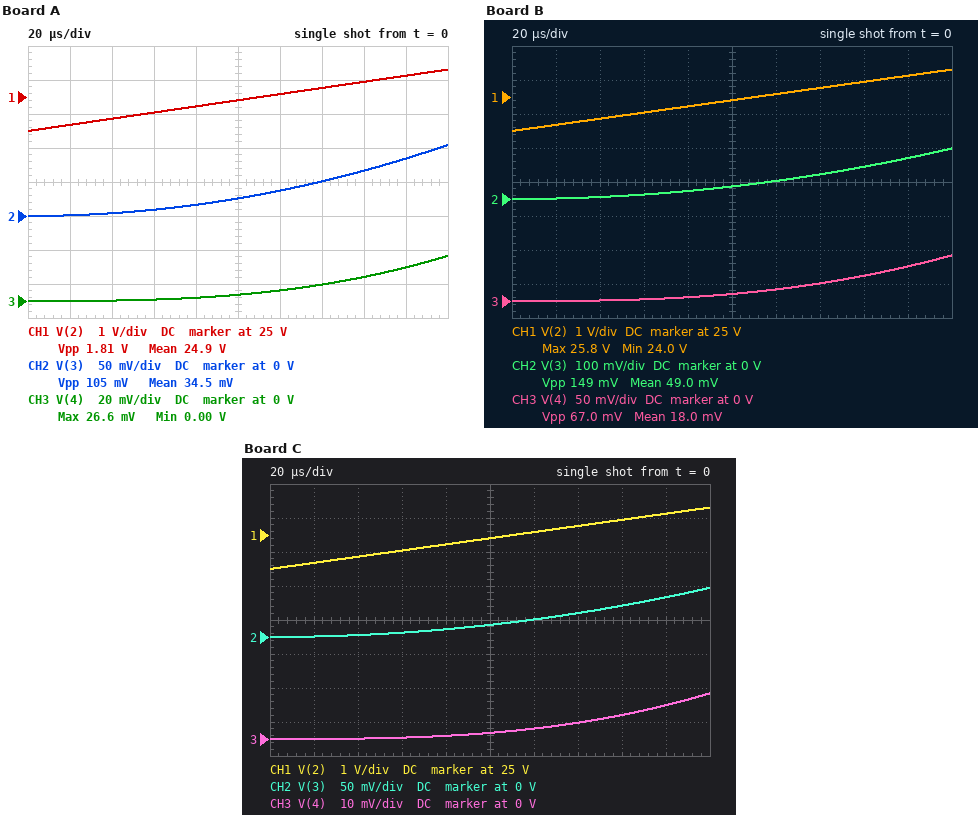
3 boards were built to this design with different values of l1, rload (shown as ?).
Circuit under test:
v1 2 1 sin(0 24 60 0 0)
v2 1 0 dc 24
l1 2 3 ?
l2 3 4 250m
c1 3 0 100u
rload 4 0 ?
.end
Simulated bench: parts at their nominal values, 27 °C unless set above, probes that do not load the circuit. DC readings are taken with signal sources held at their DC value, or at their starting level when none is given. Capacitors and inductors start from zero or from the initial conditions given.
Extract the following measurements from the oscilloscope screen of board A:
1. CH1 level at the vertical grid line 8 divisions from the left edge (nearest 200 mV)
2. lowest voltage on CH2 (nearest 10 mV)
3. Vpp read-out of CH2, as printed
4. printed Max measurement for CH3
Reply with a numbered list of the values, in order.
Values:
1. 25.4 V
2. 0 V
3. 105 mV
4. 26.6 mV
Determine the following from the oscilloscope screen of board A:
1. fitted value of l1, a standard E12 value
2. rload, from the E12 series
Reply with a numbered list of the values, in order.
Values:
1. 47 mH
2. 1.2 kΩ
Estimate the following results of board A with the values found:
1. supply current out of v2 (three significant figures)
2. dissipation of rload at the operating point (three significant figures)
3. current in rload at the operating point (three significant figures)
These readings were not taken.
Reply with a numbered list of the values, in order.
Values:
1. 20.0 mA
2. 480 mW
3. 20.0 mA
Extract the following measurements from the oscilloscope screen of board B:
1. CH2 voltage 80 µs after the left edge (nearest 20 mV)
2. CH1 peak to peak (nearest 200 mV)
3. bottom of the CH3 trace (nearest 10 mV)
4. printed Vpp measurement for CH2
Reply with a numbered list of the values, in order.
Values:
1. 20 mV
2. 1.8 V
3. 0 V
4. 149 mV
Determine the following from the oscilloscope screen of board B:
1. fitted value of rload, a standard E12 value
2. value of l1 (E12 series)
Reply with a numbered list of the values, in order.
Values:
1. 2.7 kΩ
2. 33 mH
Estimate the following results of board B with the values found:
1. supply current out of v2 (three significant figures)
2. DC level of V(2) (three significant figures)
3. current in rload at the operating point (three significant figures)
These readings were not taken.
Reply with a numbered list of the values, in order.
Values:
1. 8.89 mA
2. 24.0 V
3. 8.89 mA
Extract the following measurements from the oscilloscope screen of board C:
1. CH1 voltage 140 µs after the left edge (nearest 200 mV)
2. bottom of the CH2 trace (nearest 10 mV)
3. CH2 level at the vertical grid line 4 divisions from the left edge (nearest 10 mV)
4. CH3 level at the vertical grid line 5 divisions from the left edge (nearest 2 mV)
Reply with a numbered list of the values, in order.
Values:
1. 25.2 V
2. 0 V
3. 10 mV
4. 2 mV
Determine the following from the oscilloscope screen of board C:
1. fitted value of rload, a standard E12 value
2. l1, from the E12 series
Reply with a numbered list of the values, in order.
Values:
1. 820 Ω
2. 68 mH
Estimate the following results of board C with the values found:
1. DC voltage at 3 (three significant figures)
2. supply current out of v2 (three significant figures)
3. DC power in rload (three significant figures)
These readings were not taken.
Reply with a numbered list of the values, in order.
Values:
1. 24.0 V
2. 29.3 mA
3. 702 mW
